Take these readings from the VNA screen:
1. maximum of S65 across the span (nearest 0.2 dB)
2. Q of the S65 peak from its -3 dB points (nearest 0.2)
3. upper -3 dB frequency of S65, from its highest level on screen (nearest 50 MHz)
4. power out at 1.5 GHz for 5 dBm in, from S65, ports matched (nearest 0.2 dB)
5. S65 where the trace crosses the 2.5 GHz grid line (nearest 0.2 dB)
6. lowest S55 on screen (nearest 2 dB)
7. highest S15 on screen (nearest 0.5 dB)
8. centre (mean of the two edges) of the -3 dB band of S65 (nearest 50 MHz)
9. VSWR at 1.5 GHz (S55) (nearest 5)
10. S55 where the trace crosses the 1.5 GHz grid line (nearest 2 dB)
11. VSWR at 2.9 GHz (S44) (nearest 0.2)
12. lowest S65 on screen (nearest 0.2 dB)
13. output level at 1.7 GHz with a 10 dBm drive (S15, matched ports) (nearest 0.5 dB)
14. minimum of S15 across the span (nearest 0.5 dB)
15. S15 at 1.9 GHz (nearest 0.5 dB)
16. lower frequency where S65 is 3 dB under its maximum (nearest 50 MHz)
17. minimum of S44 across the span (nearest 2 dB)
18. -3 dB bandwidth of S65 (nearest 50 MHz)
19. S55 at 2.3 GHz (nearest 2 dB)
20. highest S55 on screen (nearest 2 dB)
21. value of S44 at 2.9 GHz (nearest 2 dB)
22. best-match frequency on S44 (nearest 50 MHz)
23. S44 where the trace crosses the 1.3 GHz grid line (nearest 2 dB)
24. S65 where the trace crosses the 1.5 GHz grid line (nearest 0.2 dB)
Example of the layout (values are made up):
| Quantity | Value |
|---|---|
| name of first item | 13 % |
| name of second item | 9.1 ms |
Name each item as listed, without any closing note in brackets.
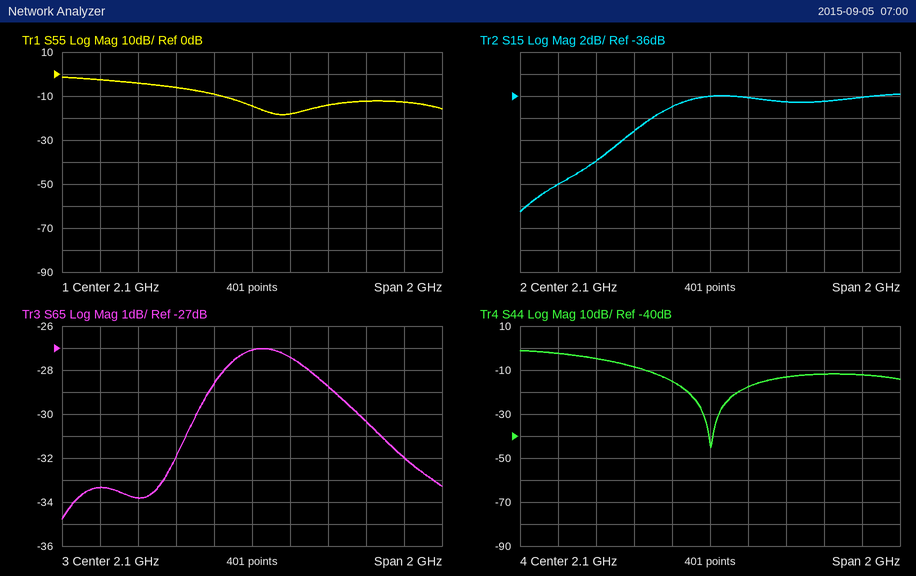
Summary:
| Quantity | Value |
|---|---|
| maximum of S65 across the span | -27.0 dB |
| Q of the S65 peak from its -3 dB points | 2.6 |
| upper -3 dB frequency of S65, from its highest level on screen | 2.65 GHz |
| power out at 1.5 GHz for 5 dBm in, from S65, ports matched | -28.8 dBm |
| S65 where the trace crosses the 2.5 GHz grid line | -28.8 dB |
| lowest S55 on screen | -18 dB |
| highest S15 on screen | -36.0 dB |
| centre (mean of the two edges) of the -3 dB band of S65 | 2.25 GHz |
| VSWR at 1.5 GHz (S55) | 5 |
| S55 where the trace crosses the 1.5 GHz grid line | -4 dB |
| VSWR at 2.9 GHz (S44) | 1.6 |
| lowest S65 on screen | -34.8 dB |
| output level at 1.7 GHz with a 10 dBm drive (S15, matched ports) | -29.0 dBm |
| minimum of S15 across the span | -46.5 dB |
| S15 at 1.9 GHz | -37.0 dB |
| lower frequency where S65 is 3 dB under its maximum | 1.80 GHz |
| minimum of S44 across the span | -46 dB |
| -3 dB bandwidth of S65 | 850 MHz |
| S55 at 2.3 GHz | -18 dB |
| highest S55 on screen | -2 dB |
| value of S44 at 2.9 GHz | -12 dB |
| best-match frequency on S44 | 2.10 GHz |
| S44 where the trace crosses the 1.3 GHz grid line | -2 dB |
| S65 where the trace crosses the 1.5 GHz grid line | -33.8 dB |
